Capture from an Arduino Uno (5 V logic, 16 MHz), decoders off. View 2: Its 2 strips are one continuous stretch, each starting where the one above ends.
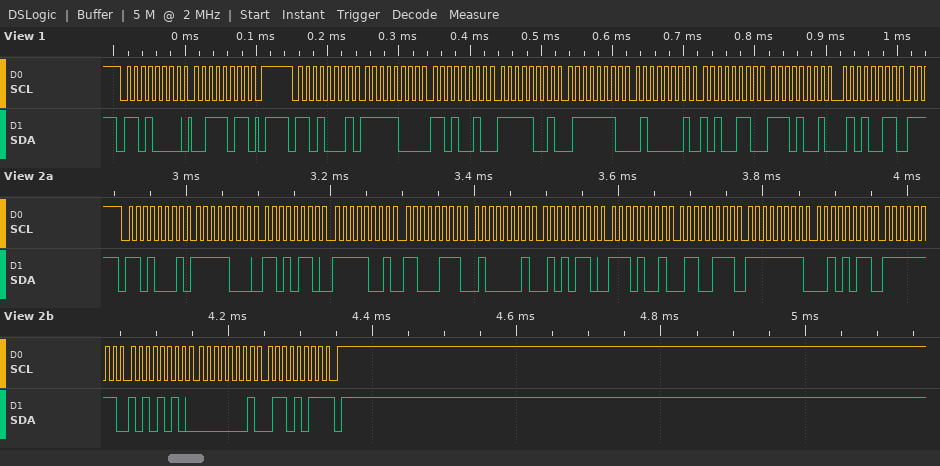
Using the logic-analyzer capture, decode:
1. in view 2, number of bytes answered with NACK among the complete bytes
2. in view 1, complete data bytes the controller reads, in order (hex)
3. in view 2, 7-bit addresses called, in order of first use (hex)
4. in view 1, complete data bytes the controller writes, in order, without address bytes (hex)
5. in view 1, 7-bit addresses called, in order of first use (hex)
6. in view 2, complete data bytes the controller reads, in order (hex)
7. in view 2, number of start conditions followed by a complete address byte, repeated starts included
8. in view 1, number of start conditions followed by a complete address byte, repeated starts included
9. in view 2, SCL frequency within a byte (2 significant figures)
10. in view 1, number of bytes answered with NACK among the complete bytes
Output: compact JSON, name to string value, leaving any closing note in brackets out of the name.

{"in view 2, number of bytes answered with NACK among the complete bytes": "1", "in view 1, complete data bytes the controller reads, in order": "F8 D2 F9 7E 41 A6 E9 53", "in view 2, 7-bit addresses called, in order of first use": "0x68", "in view 1, complete data bytes the controller writes, in order, without address bytes": "3B", "in view 1, 7-bit addresses called, in order of first use": "0x68", "in view 2, complete data bytes the controller reads, in order": "F8 D6 F9 C7 41 56 E9 67 FF 2B FF AA 01 6B", "in view 2, number of start conditions followed by a complete address byte, repeated starts included": "1", "in view 1, number of start conditions followed by a complete address byte, repeated starts included": "2", "in view 2, SCL frequency within a byte": "100 kHz", "in view 1, number of bytes answered with NACK among the complete bytes": "0"}
